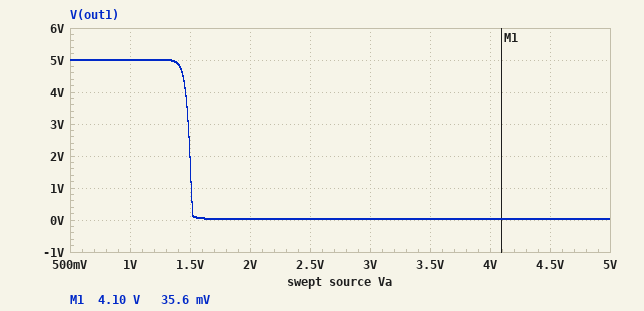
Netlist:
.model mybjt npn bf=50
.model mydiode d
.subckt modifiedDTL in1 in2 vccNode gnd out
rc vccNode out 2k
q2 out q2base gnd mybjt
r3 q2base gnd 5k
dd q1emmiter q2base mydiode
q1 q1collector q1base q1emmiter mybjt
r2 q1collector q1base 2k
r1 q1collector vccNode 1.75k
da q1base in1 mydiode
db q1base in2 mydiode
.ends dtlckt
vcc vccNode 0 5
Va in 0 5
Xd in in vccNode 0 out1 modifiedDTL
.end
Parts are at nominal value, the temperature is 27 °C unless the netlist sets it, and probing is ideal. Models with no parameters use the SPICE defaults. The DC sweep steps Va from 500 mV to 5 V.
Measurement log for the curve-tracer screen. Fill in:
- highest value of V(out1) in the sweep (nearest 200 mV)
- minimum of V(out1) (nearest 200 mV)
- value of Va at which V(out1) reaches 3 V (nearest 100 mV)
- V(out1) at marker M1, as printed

5.0 V
0 V
1.5 V
35.6 mV
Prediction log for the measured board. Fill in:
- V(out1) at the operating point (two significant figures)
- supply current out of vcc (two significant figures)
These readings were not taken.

36 mV
4.0 mA
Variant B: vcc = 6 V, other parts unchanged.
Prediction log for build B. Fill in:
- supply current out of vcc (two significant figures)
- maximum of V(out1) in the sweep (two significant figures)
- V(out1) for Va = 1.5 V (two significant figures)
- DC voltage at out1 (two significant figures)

5.1 mA
6.0 V
2.2 V
34 mV
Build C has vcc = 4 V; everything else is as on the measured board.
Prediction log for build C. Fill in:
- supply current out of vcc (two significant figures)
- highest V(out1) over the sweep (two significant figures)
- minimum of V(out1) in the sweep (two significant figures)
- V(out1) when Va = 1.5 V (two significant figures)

3.0 mA
4.0 V
40 mV
1.9 V
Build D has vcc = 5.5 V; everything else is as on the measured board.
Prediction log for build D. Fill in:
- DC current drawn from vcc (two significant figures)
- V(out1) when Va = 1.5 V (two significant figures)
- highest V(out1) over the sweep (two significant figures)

4.5 mA
2.1 V
5.5 V
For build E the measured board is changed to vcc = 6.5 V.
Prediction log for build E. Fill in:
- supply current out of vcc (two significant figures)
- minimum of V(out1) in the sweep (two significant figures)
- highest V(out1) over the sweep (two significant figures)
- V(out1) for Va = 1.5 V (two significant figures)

5.6 mA
33 mV
6.5 V
2.3 V
